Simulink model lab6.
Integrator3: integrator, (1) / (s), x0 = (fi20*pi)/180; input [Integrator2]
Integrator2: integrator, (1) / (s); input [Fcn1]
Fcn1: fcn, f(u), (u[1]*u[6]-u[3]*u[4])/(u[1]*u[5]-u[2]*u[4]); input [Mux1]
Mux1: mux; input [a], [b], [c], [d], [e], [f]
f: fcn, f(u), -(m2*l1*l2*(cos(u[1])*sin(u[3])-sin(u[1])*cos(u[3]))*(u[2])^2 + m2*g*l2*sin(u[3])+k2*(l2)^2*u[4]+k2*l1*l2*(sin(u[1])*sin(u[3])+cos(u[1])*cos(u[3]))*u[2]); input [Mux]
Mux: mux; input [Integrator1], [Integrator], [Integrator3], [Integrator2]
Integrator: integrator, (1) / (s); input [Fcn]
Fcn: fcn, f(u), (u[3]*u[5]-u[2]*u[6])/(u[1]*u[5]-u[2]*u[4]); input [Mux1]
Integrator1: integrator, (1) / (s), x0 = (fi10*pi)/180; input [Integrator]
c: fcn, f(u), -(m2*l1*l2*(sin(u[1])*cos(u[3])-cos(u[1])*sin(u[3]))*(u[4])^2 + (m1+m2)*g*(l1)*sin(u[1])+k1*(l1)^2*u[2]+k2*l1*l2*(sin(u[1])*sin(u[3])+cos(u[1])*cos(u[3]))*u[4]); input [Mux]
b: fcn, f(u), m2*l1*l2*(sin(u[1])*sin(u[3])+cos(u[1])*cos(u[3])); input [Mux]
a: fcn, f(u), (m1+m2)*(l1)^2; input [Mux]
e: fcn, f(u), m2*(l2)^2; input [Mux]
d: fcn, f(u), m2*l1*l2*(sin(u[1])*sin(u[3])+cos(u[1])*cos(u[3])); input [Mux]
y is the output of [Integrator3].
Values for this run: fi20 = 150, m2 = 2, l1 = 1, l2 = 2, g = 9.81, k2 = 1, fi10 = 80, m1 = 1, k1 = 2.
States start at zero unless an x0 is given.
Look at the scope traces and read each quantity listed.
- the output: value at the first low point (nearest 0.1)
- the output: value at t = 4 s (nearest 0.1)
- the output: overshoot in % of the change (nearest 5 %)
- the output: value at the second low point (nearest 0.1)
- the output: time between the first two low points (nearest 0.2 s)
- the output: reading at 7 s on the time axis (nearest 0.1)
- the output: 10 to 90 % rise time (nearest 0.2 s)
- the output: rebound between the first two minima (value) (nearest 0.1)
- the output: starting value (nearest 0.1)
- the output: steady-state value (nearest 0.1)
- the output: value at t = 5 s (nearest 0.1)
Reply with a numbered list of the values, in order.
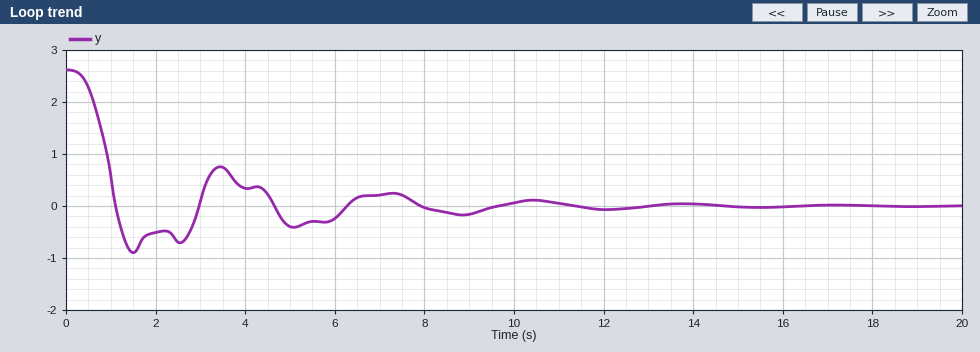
1. -0.9
2. 0.3
3. 35 %
4. -0.7
5. 1.0 s
6. 0.2
7. 0.6 s
8. -0.5
9. 2.6
10. 0.0
11. -0.4
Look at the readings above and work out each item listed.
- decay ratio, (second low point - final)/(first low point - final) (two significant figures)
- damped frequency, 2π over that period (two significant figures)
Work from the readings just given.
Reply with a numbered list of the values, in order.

1. 0.78
2. 6.3 rad/s
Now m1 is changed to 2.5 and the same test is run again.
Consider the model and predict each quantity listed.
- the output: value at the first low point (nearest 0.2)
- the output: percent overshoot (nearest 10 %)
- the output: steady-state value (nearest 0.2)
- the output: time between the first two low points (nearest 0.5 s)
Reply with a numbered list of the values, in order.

1. -1.6
2. 60 %
3. 0.0
4. 4.0 s
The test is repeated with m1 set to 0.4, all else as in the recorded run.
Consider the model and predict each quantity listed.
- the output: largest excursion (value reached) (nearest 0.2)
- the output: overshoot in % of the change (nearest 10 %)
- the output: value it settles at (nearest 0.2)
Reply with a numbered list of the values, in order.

1. -1.0
2. 40 %
3. 0.0
